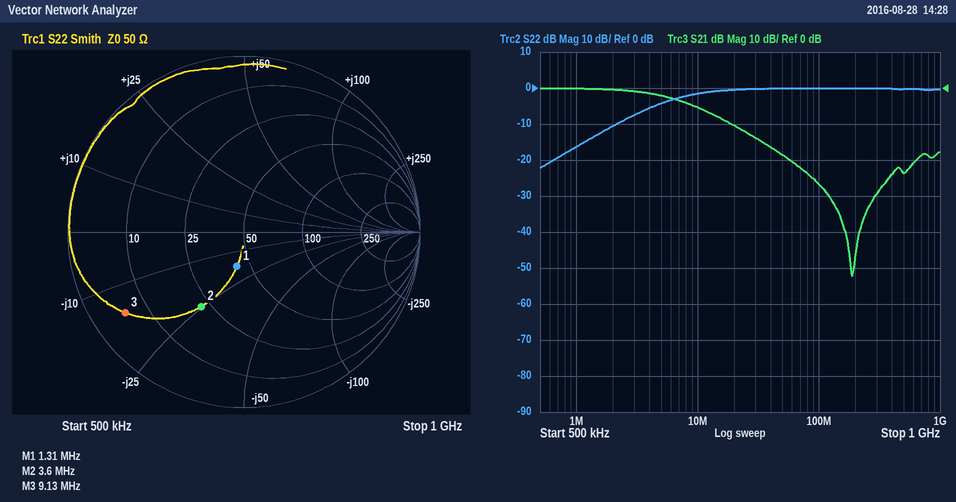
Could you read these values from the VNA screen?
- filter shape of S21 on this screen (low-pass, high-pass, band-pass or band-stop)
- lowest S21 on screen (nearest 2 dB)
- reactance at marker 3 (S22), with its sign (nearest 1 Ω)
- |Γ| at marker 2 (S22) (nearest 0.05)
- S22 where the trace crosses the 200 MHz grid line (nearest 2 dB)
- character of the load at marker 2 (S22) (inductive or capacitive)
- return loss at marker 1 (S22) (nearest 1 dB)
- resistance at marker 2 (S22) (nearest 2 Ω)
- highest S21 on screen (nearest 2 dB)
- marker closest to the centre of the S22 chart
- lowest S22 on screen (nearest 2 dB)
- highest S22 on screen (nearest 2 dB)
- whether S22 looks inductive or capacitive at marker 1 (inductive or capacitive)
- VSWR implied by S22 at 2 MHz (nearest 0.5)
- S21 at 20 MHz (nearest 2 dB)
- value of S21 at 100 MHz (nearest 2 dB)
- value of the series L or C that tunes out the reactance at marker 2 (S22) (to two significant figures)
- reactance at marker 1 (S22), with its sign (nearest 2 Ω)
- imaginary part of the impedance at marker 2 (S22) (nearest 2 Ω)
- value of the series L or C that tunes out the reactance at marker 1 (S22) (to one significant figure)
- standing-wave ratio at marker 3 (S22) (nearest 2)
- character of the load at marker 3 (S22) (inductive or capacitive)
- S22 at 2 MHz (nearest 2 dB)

low-pass
-52 dB
-15 Ω
0.50
0 dB
capacitive
14 dB
22 Ω
0 dB
marker 1
-22 dB
0 dB
capacitive
2.0
-10 dB
-26 dB
1.1 µH
-18 Ω
-24 Ω
2 µH
10
capacitive
-10 dB
